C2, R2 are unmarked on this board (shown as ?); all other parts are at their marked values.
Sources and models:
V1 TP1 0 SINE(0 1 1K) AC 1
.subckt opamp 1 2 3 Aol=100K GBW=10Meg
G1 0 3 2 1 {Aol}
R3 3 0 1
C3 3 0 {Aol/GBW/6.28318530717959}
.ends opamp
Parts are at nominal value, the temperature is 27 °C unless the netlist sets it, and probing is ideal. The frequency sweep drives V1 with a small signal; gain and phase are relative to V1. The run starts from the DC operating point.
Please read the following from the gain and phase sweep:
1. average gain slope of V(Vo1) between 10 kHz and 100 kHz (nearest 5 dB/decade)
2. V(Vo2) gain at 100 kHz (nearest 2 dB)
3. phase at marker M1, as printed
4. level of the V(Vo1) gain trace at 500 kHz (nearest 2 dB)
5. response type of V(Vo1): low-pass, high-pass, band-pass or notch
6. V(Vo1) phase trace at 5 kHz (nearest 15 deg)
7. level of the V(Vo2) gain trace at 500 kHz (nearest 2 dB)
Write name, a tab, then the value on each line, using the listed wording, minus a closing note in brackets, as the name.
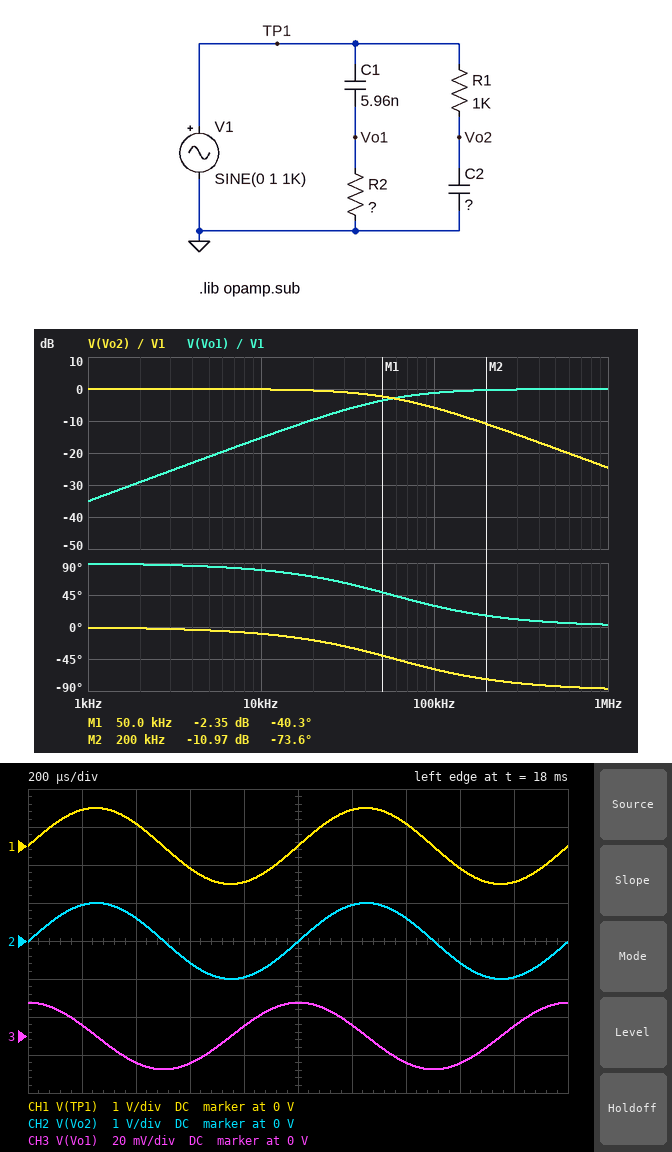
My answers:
average gain slope of V(Vo1) between 10 kHz and 100 kHz	15 dB/decade
V(Vo2) gain at 100 kHz	-6 dB
phase at marker M1, as printed	-40.3 deg
level of the V(Vo1) gain trace at 500 kHz	0 dB
response type of V(Vo1): low-pass, high-pass, band-pass or notch	high-pass
V(Vo1) phase trace at 5 kHz	90 deg
level of the V(Vo2) gain trace at 500 kHz	-18 dB
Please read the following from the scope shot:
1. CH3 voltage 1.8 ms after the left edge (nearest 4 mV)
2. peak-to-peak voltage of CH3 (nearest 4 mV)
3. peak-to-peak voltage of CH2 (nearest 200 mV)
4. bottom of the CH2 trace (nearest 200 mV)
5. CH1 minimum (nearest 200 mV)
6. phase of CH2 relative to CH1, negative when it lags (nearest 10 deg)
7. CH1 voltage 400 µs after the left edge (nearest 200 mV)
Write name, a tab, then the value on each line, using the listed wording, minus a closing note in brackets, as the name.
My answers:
CH3 voltage 1.8 ms after the left edge	4 mV
peak-to-peak voltage of CH3	36 mV
peak-to-peak voltage of CH2	2.0 V
bottom of the CH2 trace	-1.0 V
CH1 minimum	-1.0 V
phase of CH2 relative to CH1, negative when it lags	0 deg
CH1 voltage 400 µs after the left edge	600 mV
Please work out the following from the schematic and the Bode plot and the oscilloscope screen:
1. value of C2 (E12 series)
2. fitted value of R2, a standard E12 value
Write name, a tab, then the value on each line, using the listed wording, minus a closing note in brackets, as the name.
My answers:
value of C2	2.7 nF
fitted value of R2, a standard E12 value	470 Ω
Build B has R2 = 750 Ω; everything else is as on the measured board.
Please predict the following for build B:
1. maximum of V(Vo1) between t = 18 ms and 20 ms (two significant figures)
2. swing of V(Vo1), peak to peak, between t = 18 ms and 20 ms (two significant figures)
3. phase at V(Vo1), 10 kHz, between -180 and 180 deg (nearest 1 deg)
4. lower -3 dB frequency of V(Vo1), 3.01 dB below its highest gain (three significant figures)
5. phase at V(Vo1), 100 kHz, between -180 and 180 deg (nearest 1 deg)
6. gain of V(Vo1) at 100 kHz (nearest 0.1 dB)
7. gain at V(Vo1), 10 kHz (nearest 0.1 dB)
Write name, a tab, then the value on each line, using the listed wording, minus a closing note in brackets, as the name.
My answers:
maximum of V(Vo1) between t = 18 ms and 20 ms	28 mV
swing of V(Vo1), peak to peak, between t = 18 ms and 20 ms	56 mV
phase at V(Vo1), 10 kHz, between -180 and 180 deg	74 deg
lower -3 dB frequency of V(Vo1), 3.01 dB below its highest gain	35.6 kHz
phase at V(Vo1), 100 kHz, between -180 and 180 deg	20 deg
gain of V(Vo1) at 100 kHz	-0.5 dB
gain at V(Vo1), 10 kHz	-11.4 dB
